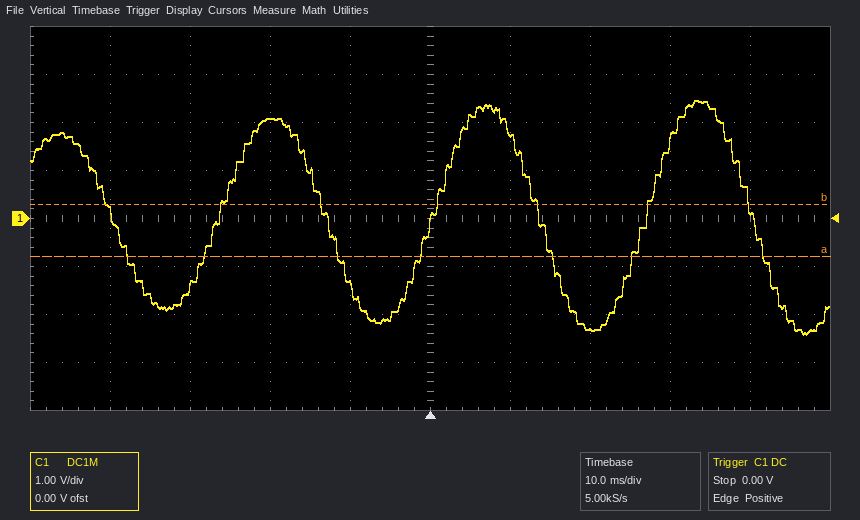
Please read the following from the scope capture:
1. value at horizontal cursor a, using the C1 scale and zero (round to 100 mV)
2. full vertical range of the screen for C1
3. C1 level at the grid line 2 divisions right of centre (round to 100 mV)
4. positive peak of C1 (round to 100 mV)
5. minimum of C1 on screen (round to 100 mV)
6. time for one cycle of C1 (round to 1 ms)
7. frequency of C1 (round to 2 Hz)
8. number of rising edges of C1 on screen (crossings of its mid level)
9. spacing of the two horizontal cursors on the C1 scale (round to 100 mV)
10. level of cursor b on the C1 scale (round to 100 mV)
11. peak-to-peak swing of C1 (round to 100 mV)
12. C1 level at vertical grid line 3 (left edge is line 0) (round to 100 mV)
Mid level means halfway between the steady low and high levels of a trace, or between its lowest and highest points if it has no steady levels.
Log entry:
-800 mV
8 V
-2.3 V
2.5 V
-2.4 V
27 ms
38 Hz
3
1.1 V
300 mV
4.9 V
2.1 V
